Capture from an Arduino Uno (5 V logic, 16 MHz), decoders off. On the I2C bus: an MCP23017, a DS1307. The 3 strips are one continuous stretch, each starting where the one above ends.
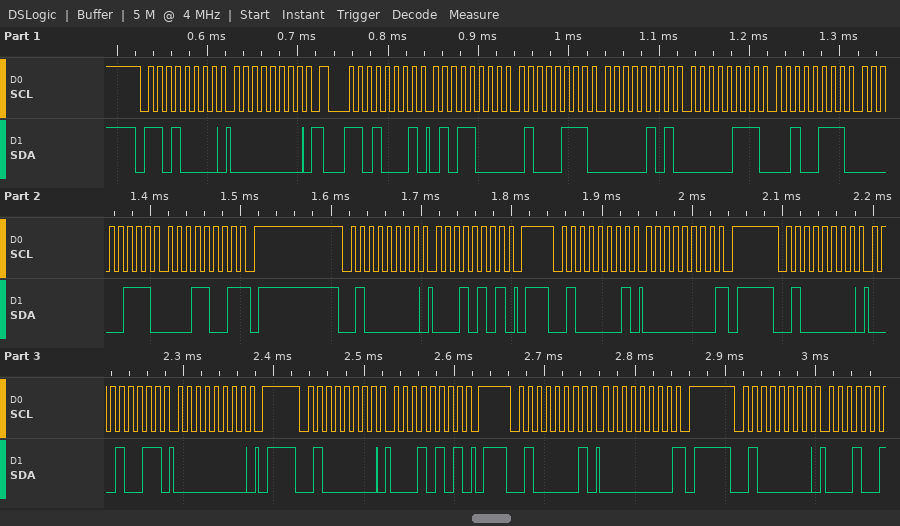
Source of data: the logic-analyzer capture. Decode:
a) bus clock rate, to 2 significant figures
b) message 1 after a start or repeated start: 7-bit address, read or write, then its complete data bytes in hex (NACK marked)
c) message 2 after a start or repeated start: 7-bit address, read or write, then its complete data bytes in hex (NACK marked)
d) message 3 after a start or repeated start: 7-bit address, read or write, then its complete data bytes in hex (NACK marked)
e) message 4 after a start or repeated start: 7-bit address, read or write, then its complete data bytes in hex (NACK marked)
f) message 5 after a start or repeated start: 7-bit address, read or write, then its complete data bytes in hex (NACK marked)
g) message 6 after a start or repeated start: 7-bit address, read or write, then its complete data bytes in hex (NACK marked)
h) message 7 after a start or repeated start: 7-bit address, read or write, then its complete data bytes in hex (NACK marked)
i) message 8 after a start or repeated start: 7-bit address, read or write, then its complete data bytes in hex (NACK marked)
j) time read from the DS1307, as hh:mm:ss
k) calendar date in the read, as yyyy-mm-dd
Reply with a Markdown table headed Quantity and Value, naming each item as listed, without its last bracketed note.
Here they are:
| Quantity | Value |
|---|---|
| bus clock rate, to 2 significant figures | 100 kHz |
| message 1 after a start or repeated start: 7-bit address, read or write, then its complete data bytes in hex | 0x68 write: 00 |
| message 2 after a start or repeated start: 7-bit address, read or write, then its complete data bytes in hex | 0x68 read: 58 47 05 07 27 07 19 NACK |
| message 3 after a start or repeated start: 7-bit address, read or write, then its complete data bytes in hex | 0x20 write: 15 |
| message 4 after a start or repeated start: 7-bit address, read or write, then its complete data bytes in hex | 0x20 read: 00 NACK |
| message 5 after a start or repeated start: 7-bit address, read or write, then its complete data bytes in hex | 0x20 write: 13 00 |
| message 6 after a start or repeated start: 7-bit address, read or write, then its complete data bytes in hex | 0x20 write: 15 |
| message 7 after a start or repeated start: 7-bit address, read or write, then its complete data bytes in hex | 0x20 read: 00 NACK |
| message 8 after a start or repeated start: 7-bit address, read or write, then its complete data bytes in hex | 0x20 write |
| time read from the DS1307, as hh:mm:ss | 05:47:58 |
| calendar date in the read, as yyyy-mm-dd | 2019-07-27 |
